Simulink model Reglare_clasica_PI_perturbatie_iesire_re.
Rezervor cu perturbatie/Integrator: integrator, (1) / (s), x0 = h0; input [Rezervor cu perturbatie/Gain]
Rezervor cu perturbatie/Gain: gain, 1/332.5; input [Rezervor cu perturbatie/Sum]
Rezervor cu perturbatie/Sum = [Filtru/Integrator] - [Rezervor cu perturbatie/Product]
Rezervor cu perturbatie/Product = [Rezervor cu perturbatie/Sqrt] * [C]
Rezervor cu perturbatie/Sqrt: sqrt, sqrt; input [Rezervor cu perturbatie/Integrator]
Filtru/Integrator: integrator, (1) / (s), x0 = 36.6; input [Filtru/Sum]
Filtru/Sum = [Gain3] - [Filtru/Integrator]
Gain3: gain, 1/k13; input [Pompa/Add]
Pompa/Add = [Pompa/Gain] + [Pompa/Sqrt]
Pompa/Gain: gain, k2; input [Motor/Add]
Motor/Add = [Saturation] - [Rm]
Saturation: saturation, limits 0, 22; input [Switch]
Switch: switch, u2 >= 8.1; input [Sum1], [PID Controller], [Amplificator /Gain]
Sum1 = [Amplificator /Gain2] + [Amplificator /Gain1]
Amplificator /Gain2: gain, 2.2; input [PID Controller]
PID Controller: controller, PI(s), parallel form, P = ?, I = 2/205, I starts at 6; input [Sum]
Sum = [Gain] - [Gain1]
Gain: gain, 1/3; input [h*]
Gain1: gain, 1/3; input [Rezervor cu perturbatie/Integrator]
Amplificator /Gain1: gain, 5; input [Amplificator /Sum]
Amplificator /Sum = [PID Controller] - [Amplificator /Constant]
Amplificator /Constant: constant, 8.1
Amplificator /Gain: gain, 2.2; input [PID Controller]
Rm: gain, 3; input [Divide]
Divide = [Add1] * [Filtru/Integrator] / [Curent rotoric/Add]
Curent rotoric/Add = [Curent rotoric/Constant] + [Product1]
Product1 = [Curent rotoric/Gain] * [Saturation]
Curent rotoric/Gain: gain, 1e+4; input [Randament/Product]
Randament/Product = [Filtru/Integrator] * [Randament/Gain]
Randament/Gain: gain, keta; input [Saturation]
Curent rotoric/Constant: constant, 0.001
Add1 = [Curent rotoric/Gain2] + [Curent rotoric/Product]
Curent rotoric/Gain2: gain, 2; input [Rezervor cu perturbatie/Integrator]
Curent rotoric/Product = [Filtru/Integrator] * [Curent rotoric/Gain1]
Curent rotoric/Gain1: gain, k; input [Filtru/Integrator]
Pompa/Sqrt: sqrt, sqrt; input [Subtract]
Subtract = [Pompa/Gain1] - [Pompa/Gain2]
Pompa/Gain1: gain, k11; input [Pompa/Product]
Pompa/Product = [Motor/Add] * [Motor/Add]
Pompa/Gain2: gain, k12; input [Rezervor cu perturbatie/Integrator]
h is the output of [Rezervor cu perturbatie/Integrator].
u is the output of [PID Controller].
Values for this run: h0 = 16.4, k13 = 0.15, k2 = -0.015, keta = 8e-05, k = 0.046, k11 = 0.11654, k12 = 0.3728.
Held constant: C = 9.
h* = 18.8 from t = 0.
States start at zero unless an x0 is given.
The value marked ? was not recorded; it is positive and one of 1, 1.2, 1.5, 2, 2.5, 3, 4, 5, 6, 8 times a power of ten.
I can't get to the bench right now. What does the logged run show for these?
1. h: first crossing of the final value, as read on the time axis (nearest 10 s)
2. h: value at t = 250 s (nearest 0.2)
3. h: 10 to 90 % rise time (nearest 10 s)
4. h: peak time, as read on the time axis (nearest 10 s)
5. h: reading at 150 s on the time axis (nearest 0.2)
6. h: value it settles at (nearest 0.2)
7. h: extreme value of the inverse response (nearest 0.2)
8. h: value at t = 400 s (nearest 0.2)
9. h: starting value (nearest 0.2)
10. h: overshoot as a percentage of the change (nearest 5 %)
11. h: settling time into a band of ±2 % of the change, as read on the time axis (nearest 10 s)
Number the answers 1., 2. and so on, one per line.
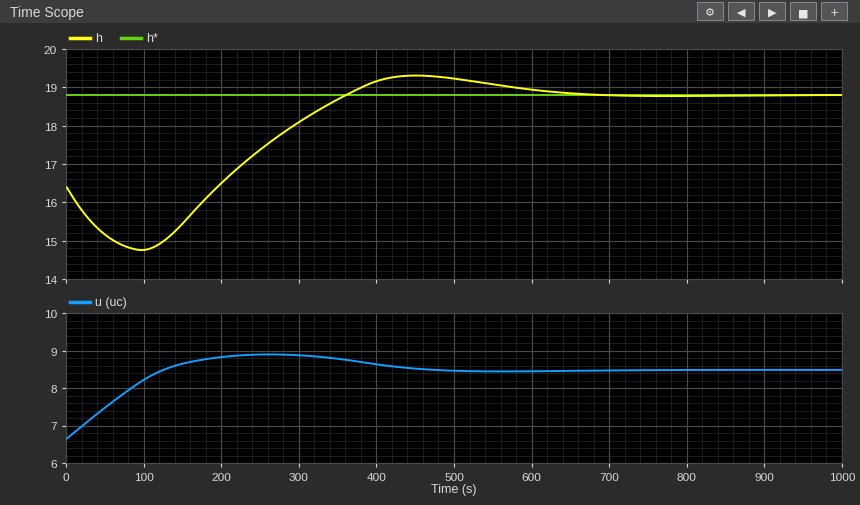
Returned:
1. 360 s
2. 17.4
3. 130 s
4. 450 s
5. 15.4
6. 18.8
7. 14.8
8. 19.2
9. 16.4
10. 20 %
11. 650 s
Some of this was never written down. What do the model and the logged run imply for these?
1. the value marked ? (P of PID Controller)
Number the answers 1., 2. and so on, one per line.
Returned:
1. 0.8
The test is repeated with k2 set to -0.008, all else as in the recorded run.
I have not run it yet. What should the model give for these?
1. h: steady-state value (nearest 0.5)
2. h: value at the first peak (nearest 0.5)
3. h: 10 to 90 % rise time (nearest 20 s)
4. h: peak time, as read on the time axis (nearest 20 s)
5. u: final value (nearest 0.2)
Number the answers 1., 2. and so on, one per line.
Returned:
1. 19.0
2. 19.0
3. 120 s
4. 420 s
5. 8.4
